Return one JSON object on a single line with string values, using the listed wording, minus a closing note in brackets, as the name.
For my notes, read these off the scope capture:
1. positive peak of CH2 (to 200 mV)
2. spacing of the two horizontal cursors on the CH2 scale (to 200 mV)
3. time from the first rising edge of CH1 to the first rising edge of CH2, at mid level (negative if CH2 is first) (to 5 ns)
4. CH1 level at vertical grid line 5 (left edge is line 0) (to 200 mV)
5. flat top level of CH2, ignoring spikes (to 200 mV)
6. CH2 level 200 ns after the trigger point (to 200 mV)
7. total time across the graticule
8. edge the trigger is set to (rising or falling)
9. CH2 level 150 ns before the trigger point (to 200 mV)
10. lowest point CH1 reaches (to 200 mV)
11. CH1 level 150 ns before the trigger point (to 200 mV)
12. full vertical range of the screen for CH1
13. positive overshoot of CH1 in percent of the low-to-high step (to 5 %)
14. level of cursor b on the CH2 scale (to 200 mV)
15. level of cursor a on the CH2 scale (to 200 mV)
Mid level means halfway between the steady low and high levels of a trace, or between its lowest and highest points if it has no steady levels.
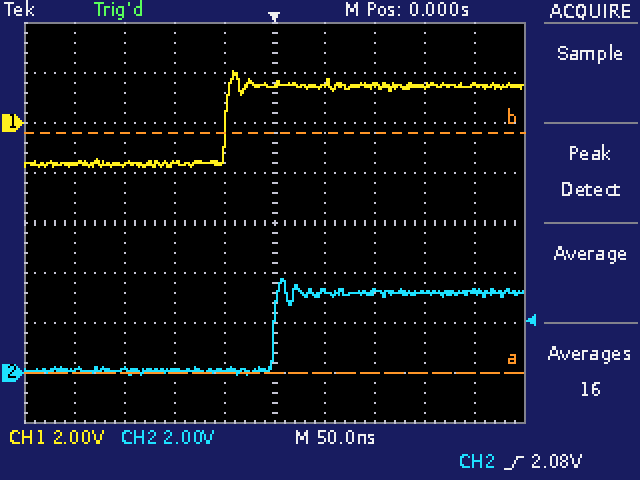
{"positive peak of CH2": "3.8 V", "spacing of the two horizontal cursors on the CH2 scale": "9.6 V", "time from the first rising edge of CH1 to the first rising edge of CH2, at mid level (negative if CH2 is first)": "+50 ns", "CH1 level at vertical grid line 5 (left edge is line 0)": "1.6 V", "flat top level of CH2, ignoring spikes": "3.2 V", "CH2 level 200 ns after the trigger point": "3.2 V", "total time across the graticule": "500 ns", "edge the trigger is set to": "rising", "CH2 level 150 ns before the trigger point": "200 mV", "lowest point CH1 reaches": "-1.8 V", "CH1 level 150 ns before the trigger point": "-1.6 V", "full vertical range of the screen for CH1": "16 V", "positive overshoot of CH1 in percent of the low-to-high step": "20 %", "level of cursor b on the CH2 scale": "9.6 V", "level of cursor a on the CH2 scale": "0.0 V"}
